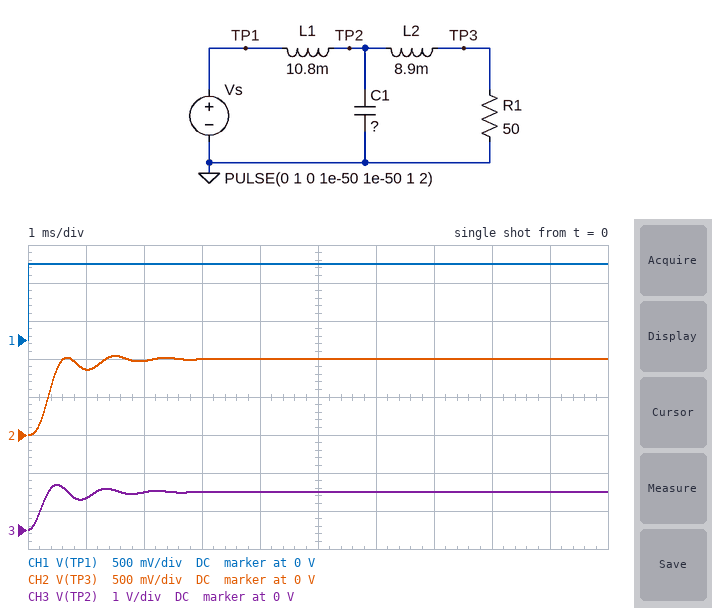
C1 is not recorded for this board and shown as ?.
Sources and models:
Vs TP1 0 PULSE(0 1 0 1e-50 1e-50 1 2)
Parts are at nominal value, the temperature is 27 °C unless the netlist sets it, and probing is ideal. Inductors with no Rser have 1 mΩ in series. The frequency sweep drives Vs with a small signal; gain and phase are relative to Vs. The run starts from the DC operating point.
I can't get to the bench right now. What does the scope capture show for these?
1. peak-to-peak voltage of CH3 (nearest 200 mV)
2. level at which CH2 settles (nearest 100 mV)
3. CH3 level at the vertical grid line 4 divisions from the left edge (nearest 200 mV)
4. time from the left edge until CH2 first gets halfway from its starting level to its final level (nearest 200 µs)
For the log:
1.2 V
1.0 V
1.0 V
400 µs
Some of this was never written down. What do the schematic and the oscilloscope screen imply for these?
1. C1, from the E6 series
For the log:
3.3 µF
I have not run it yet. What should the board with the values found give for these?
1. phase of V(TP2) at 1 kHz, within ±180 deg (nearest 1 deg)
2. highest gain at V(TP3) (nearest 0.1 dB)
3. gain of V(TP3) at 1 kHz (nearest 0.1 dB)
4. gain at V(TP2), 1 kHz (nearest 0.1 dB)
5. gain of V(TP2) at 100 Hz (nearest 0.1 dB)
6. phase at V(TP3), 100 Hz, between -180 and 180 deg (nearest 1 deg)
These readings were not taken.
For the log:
-66 deg
0.5 dB
0.1 dB
3.6 dB
-0.1 dB
-14 deg
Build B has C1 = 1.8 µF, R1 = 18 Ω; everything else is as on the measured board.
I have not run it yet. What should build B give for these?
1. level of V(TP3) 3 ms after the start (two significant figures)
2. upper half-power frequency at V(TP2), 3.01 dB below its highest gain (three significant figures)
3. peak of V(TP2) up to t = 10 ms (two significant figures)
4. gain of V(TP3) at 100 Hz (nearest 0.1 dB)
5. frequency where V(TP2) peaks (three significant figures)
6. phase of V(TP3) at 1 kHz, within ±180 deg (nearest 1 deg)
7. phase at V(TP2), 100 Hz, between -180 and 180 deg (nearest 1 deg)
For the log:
930 mV
1.77 kHz
1.1 V
-1.6 dB
1.69 kHz
-87 deg
-17 deg
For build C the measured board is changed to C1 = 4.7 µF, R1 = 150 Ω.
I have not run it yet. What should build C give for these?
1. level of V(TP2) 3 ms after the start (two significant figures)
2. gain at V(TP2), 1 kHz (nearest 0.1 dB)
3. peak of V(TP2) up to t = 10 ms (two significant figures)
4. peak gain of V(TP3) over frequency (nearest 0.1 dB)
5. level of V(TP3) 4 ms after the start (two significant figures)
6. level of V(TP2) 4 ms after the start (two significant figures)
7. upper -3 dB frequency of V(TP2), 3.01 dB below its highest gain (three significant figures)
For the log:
940 mV
0.5 dB
1.6 V
10.0 dB
970 mV
960 mV
828 Hz
